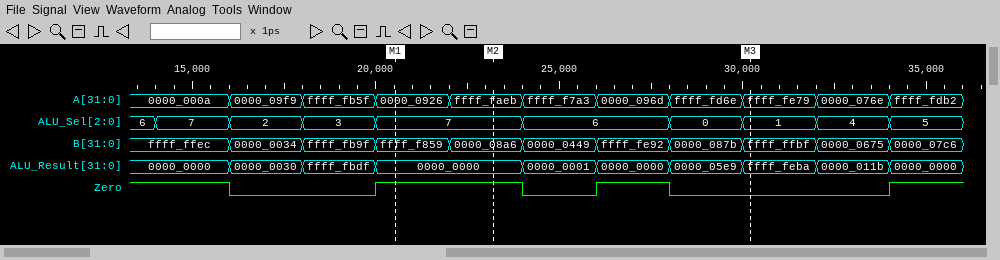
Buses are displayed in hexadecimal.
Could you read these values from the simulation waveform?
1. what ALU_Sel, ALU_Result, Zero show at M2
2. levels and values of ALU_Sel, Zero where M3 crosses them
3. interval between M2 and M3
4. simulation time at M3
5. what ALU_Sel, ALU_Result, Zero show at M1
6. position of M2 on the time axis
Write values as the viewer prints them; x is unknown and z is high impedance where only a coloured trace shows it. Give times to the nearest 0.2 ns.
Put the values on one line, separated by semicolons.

ALU_Sel=7, ALU_Result=0000_0000, Zero=1; ALU_Sel=1, Zero=0; 7 ns; 30.2 ns; ALU_Sel=7, ALU_Result=0000_0000, Zero=1; 23.2 ns
